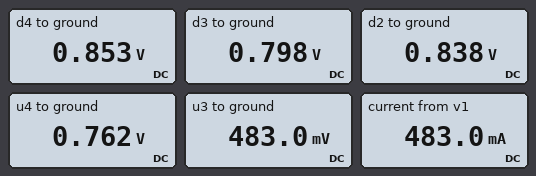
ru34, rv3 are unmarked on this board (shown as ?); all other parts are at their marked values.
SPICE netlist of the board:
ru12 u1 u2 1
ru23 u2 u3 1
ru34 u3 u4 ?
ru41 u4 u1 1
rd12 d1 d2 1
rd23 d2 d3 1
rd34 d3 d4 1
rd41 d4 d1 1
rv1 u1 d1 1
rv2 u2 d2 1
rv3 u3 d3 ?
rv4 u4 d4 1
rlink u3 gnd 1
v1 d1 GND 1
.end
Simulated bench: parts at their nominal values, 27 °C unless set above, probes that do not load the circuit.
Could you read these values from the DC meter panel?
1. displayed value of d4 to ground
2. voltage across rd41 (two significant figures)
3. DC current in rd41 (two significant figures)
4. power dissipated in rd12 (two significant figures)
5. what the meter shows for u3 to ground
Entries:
0.853 V
150 mV
150 mA
26 mW
483.0 mV
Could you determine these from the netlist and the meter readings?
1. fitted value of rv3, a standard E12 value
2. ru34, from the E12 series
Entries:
3.3 Ω
1.8 Ω
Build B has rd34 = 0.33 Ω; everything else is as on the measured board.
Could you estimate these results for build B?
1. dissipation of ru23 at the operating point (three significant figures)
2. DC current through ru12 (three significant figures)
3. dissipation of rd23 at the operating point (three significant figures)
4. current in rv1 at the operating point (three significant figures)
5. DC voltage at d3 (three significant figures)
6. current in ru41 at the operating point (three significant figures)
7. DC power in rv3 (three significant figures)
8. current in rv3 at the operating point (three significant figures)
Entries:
54.5 mW
107 mA
755 µW
174 mA
818 mV
67.4 mA
33.5 mW
101 mA
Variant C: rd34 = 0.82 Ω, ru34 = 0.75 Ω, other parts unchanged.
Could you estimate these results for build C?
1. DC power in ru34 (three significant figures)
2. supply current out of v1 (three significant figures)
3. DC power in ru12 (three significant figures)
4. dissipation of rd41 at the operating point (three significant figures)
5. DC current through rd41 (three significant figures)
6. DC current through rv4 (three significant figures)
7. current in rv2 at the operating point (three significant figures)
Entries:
42.3 mW
522 mA
7.14 mW
28.9 mW
170 mA
130 mA
117 mA
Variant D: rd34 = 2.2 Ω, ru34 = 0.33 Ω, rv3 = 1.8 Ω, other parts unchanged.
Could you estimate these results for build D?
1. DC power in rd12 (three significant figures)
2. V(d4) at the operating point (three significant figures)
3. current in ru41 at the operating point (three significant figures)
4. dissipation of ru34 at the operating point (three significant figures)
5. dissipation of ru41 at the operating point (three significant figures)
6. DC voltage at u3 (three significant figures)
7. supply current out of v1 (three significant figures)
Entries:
30.1 mW
815 mV
137 mA
28.2 mW
18.7 mW
563 mV
563 mA
